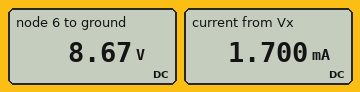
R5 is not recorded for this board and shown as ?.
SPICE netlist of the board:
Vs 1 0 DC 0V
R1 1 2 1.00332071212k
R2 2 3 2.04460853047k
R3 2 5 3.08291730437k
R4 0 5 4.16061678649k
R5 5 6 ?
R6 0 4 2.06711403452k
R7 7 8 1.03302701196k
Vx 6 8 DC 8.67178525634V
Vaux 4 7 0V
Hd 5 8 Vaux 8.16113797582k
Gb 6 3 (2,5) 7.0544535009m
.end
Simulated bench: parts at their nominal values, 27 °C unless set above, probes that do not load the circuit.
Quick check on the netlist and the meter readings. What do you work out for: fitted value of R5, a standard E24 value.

5.1 kΩ
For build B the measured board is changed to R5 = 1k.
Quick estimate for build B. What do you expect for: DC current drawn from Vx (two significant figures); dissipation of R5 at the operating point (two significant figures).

8.7 mA
75 mW
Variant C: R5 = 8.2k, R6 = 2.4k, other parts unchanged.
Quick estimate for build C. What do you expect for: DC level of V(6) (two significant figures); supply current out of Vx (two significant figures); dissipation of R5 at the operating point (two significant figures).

8.7 V
1.1 mA
9.2 mW
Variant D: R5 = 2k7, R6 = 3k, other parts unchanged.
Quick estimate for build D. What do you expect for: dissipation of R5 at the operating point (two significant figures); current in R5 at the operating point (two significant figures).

28 mW
3.2 mA
